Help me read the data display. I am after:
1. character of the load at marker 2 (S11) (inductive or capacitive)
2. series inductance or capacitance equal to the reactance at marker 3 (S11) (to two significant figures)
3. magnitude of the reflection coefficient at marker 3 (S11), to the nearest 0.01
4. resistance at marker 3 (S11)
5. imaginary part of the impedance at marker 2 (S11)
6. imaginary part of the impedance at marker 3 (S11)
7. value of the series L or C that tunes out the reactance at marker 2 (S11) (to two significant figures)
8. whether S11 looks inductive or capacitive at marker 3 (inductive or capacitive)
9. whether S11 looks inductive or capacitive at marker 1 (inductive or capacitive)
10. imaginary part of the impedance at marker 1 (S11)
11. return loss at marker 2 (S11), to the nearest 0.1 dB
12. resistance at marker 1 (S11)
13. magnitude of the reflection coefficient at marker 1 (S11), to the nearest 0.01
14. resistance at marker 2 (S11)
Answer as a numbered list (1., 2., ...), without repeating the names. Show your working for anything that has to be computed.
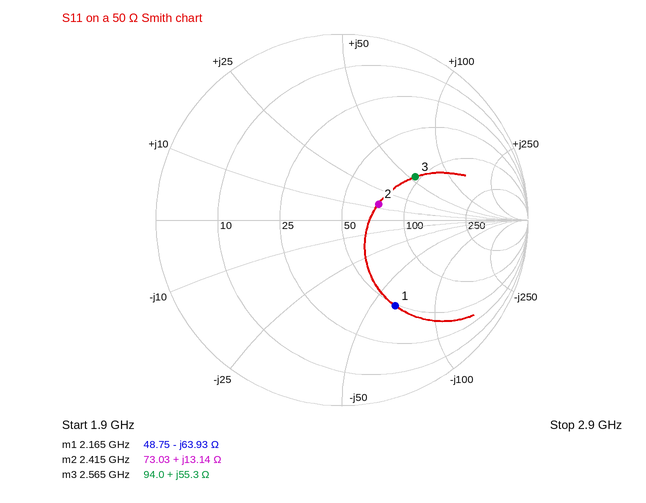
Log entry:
1. inductive
2. L = 55.3 Ω/(2π × 2.565 GHz) ≈ 3.4 nH
3. 0.46
4. 94.0 Ω
5. +13.14 Ω
6. +55.3 Ω
7. C = 1/(2π × 2.415 GHz × 13.14 Ω) ≈ 5.0 pF
8. inductive
9. capacitive
10. -63.93 Ω
11. 13.4 dB
12. 48.75 Ω
13. 0.54
14. 73.03 Ω
